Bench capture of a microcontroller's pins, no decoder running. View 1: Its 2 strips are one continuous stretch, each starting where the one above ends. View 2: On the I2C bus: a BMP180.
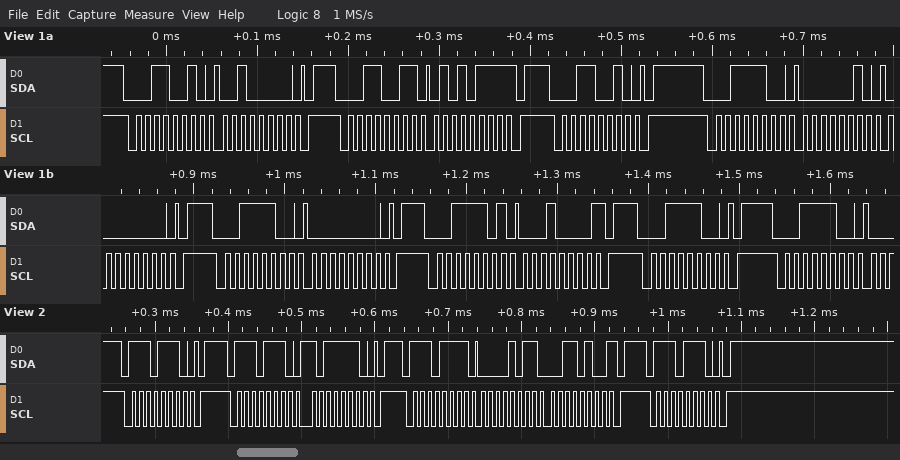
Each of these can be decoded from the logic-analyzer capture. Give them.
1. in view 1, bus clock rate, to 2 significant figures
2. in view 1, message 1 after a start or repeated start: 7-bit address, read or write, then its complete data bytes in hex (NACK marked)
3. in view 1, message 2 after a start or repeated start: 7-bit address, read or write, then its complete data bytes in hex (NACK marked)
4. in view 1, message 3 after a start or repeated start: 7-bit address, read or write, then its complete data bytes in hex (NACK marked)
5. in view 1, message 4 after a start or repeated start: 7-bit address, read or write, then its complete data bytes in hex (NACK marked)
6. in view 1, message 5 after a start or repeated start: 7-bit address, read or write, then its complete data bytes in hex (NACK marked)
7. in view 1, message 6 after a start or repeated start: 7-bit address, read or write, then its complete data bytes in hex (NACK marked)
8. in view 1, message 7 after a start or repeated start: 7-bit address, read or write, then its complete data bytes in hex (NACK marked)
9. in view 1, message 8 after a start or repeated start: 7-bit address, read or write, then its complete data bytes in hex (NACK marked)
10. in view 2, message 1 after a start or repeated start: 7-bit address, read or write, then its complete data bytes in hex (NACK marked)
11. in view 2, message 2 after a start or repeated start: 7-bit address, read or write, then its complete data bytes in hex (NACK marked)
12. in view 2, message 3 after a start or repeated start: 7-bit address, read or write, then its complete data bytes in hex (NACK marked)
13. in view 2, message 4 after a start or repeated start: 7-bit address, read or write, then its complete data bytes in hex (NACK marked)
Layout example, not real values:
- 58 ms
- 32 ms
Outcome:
- 100 kHz
- 0x19 write: 20
- 0x19 read: 57 NACK
- 0x19 write
- 0x1E write: 02 00
- 0x1E write: 00
- 0x1E read: 10 NACK
- 0x1E write
- 0x1E write
- 0x77 write
- 0x77 write: BE
- 0x77 read: 0B 34 NACK
- 0x77 write
